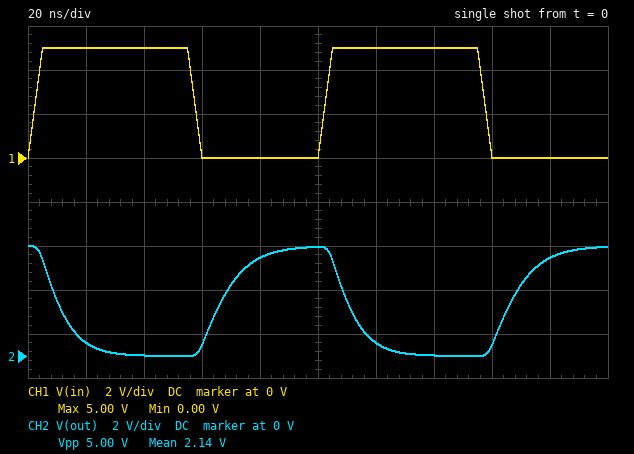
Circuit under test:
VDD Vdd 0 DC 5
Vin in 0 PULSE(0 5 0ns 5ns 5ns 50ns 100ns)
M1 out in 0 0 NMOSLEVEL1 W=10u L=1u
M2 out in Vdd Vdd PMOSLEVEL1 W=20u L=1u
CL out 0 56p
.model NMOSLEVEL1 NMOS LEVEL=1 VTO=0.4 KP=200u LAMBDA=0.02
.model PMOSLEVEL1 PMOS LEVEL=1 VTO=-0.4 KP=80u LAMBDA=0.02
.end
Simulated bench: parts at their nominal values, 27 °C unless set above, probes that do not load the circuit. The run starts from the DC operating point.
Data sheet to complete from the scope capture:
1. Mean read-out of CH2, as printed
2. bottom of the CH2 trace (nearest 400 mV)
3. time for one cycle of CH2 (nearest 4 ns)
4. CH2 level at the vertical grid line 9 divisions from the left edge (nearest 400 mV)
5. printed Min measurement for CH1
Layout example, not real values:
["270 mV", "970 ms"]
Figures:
["2.14 V", "0 V", "100 ns", "4.4 V", "0.00 V"]
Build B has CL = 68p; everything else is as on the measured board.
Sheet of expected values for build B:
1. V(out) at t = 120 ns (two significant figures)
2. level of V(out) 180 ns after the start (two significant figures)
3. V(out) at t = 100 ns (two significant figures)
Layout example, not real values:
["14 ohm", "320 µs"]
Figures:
["910 mV", "4.1 V", "4.9 V"]
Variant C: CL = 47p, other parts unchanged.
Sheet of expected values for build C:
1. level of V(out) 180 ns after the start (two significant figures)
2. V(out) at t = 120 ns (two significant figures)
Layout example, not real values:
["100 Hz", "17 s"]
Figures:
["4.7 V", "360 mV"]
